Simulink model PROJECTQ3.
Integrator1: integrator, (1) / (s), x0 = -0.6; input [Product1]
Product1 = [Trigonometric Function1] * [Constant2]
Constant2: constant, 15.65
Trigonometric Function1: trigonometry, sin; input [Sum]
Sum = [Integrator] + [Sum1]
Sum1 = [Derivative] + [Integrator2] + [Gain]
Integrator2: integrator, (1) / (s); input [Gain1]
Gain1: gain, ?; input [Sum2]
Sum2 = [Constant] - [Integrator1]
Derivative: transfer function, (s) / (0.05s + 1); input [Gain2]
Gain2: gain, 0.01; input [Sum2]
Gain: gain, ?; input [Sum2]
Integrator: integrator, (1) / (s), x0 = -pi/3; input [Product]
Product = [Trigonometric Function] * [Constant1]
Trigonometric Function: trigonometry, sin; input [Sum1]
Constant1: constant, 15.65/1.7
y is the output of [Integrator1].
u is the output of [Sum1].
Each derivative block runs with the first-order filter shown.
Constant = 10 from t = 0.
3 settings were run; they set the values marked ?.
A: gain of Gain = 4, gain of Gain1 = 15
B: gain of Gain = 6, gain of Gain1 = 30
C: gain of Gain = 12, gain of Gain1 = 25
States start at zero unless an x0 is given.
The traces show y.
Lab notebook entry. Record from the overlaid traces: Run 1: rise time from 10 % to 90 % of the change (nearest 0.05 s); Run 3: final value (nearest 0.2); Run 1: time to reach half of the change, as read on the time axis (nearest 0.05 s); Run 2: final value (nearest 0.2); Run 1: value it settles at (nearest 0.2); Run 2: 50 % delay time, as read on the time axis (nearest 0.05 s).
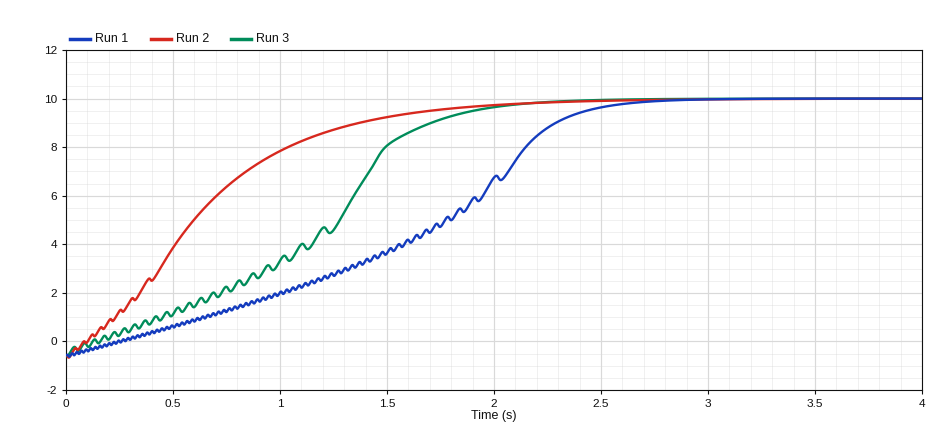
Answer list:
1.85 s
10.0
1.70 s
10.0
10.0
0.55 s
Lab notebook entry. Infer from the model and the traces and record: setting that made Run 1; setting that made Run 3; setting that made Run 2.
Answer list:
B
A
C
